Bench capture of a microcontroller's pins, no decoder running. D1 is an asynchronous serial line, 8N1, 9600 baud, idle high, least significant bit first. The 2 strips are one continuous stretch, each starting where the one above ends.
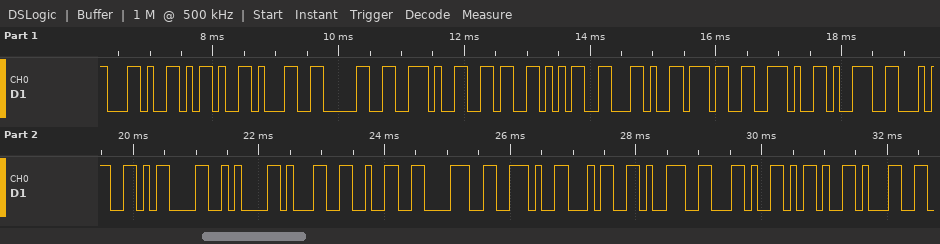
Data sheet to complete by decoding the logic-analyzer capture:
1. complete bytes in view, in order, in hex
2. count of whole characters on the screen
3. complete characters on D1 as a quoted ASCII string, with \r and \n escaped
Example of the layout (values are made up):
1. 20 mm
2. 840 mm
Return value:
1. 0x2C 0x2D 0x31 0x30 0x2E 0x36 0x35 0x2C 0x37 0x2E 0x39 0x34 0x0D 0x0A 0x31 0x32 0x38 0x2E 0x34 0x39 0x2C 0x2D 0x31
2. 23
3. ",-10.65,7.94\r\n128.49,-1"
